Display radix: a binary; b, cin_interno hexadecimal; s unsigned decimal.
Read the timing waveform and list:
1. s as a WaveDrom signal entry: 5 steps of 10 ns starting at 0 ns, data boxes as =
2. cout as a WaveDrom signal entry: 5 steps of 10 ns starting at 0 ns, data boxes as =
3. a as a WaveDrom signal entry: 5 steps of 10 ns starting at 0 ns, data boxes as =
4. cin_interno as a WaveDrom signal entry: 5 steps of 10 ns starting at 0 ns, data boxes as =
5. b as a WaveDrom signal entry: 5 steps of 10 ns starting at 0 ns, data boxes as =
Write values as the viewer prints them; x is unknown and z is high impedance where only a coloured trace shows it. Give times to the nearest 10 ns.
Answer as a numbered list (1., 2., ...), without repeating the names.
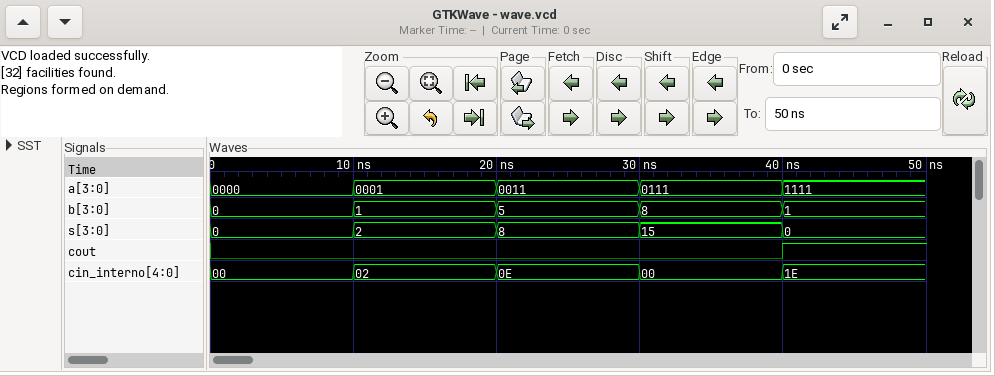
1. {name: 's', wave: '=====', data: '0 2 8 15 0'}
2. {name: 'cout', wave: '0...1'}
3. {name: 'a', wave: '=====', data: '0000 0001 0011 0111 1111'}
4. {name: 'cin_interno', wave: '=====', data: '00 02 0E 00 1E'}
5. {name: 'b', wave: '=====', data: '0 1 5 8 1'}
